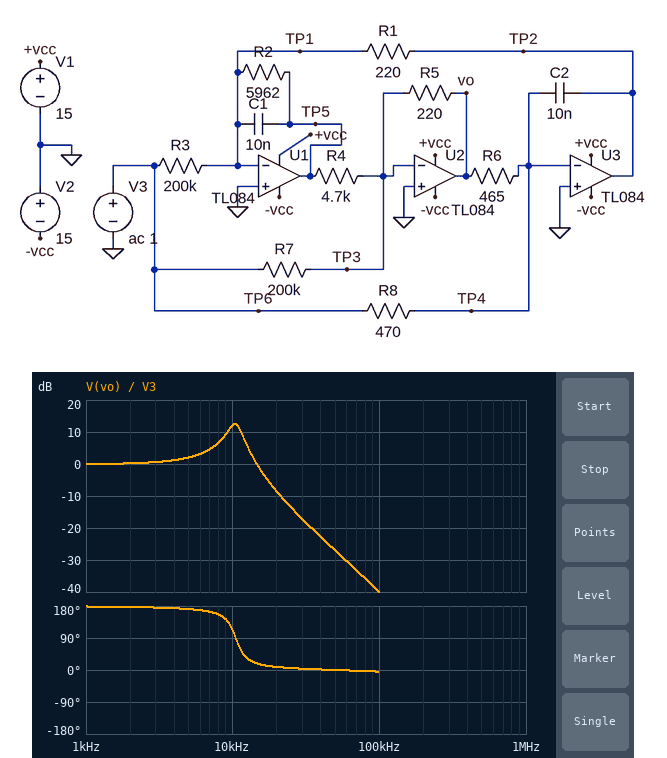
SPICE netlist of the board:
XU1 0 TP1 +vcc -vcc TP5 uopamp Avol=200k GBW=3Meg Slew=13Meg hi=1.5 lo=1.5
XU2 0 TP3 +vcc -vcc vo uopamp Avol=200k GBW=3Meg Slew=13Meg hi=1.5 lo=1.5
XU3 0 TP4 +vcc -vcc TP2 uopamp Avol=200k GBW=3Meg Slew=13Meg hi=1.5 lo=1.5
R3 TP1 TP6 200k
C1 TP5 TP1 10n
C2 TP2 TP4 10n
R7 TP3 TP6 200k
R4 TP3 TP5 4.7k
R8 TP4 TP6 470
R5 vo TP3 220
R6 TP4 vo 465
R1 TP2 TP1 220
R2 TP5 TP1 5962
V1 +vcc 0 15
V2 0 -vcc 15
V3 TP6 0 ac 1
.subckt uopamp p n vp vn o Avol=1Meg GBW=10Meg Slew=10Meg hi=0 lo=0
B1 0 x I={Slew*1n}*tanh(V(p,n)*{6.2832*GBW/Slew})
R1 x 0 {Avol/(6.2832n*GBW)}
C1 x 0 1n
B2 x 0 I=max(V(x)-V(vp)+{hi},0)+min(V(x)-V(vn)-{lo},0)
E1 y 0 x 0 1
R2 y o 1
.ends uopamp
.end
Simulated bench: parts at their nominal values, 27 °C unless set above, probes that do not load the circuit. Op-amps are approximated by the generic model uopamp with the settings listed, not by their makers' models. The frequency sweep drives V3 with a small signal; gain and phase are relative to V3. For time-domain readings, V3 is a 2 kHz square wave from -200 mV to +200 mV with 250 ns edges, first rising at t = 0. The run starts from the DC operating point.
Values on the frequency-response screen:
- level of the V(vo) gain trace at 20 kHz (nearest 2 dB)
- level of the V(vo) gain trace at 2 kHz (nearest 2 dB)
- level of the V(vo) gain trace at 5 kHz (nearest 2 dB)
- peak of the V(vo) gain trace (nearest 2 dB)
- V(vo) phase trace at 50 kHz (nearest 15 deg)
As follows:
-8 dB
0 dB
2 dB
12 dB
0 deg
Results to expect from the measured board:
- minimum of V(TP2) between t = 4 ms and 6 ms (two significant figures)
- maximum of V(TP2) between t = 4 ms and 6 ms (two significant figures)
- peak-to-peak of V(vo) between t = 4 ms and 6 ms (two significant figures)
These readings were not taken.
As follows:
-1.3 V
1.3 V
1.0 V
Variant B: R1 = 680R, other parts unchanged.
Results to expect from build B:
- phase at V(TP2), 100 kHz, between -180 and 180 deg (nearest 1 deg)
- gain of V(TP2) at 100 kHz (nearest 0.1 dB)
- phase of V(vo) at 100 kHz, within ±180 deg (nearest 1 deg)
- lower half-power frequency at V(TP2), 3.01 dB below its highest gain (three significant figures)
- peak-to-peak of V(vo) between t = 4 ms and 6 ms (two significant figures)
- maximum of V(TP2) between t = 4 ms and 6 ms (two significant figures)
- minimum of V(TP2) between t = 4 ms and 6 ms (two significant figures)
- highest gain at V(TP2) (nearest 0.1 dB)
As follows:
88 deg
-9.6 dB
-6 deg
4.77 kHz
840 mV
2.2 V
-2.2 V
22.8 dB
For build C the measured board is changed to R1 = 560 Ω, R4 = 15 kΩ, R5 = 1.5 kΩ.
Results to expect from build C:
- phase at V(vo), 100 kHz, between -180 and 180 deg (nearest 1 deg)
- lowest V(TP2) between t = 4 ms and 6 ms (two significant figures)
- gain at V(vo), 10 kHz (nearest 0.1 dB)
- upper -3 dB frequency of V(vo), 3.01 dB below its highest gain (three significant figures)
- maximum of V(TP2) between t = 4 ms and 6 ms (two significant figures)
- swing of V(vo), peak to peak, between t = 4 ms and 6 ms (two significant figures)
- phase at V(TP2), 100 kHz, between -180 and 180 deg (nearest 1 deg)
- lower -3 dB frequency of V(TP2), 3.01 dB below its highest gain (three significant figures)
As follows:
-16 deg
-1.4 V
11.0 dB
10.7 kHz
1.4 V
970 mV
88 deg
8.49 kHz
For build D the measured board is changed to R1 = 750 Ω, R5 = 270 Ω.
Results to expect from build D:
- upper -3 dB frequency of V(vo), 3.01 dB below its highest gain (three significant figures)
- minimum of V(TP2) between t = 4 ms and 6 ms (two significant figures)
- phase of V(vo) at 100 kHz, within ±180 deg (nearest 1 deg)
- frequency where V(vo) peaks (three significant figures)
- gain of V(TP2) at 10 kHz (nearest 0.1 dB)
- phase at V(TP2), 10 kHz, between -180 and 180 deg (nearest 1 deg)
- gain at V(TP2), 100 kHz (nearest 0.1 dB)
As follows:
7.30 kHz
-2.1 V
-6 deg
6.09 kHz
14.4 dB
99 deg
-9.6 dB
